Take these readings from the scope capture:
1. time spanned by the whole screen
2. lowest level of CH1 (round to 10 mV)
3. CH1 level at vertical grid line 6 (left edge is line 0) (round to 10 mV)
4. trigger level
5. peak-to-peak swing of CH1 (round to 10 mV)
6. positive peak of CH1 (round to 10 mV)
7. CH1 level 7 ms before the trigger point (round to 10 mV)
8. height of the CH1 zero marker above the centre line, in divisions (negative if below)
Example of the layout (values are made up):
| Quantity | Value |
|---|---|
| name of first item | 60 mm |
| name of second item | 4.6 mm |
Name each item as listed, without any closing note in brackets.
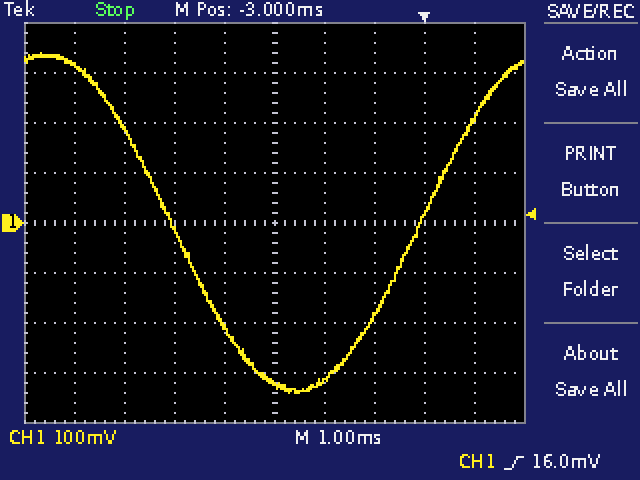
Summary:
| Quantity | Value |
|---|---|
| time spanned by the whole screen | 10 ms |
| lowest level of CH1 | -340 mV |
| CH1 level at vertical grid line 6 (left edge is line 0) | -320 mV |
| trigger level | 16.0 mV |
| peak-to-peak swing of CH1 | 680 mV |
| positive peak of CH1 | 340 mV |
| CH1 level 7 ms before the trigger point | 320 mV |
| height of the CH1 zero marker above the centre line, in divisions | 0.0 div |
